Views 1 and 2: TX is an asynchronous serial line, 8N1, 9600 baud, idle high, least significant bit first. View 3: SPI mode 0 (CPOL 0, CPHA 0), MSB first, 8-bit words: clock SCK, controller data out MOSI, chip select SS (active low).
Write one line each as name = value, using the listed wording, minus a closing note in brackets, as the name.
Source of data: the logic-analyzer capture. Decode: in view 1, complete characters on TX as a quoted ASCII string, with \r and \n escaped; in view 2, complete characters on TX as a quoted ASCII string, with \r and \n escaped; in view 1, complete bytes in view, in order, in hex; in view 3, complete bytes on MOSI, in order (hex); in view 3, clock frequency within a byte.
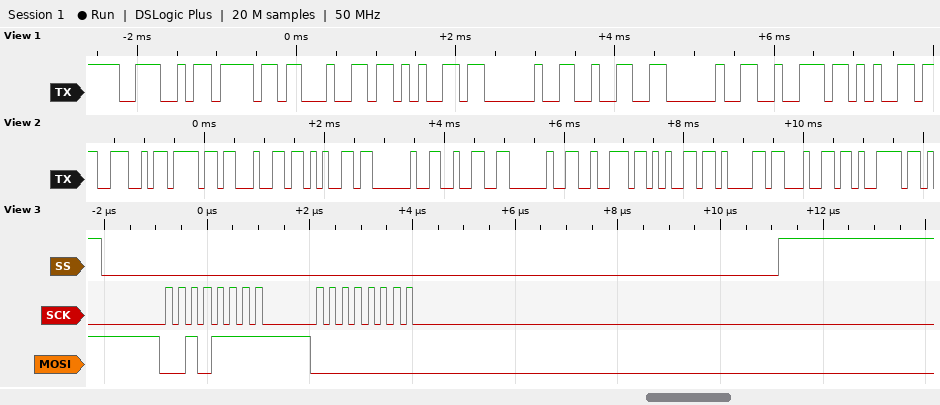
in view 1, complete characters on TX as a quoted ASCII string, with \r and \n escaped = "Node 2 re"
in view 2, complete characters on TX as a quoted ASCII string, with \r and \n escaped = "Node 2 ready"
in view 1, complete bytes in view, in order, in hex = 4E 6F 64 65 20 32 20 72 65
in view 3, complete bytes on MOSI, in order = 2F 00
in view 3, clock frequency within a byte = 4 MHz
